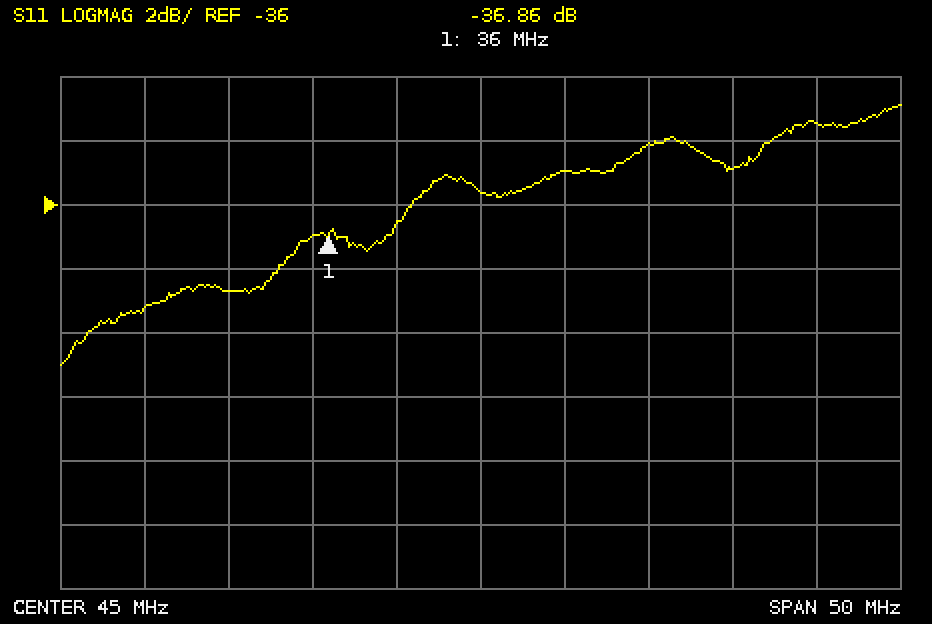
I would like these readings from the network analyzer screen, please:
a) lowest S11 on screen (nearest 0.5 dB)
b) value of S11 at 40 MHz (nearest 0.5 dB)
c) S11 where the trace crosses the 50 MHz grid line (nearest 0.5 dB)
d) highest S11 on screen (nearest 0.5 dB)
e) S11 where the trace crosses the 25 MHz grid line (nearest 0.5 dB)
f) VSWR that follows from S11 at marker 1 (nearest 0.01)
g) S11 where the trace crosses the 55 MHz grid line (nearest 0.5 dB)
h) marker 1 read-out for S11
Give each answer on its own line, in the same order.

-41.0 dB
-36.5 dB
-35.0 dB
-33.0 dB
-39.0 dB
1.03
-34.0 dB
-36.86 dB
